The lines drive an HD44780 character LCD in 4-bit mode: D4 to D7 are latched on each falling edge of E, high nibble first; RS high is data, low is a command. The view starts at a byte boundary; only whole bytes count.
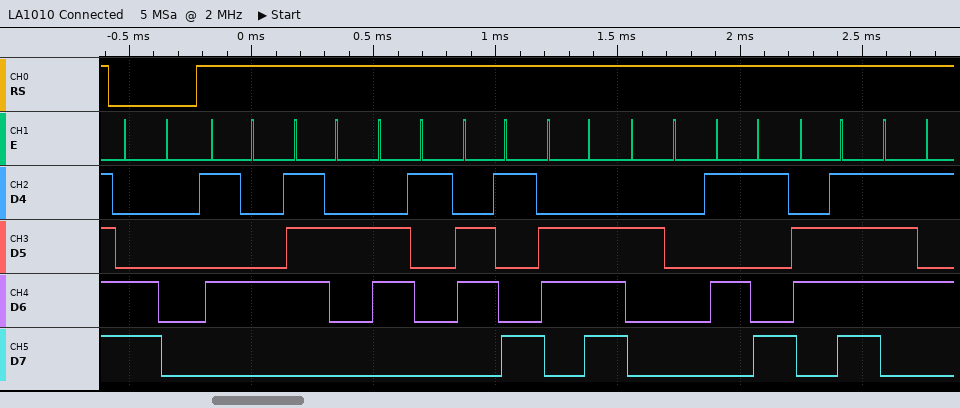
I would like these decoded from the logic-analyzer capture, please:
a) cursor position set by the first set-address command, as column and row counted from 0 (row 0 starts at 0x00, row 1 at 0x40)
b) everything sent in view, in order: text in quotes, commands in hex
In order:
column 0, row 1
0xC0 "Train You"
